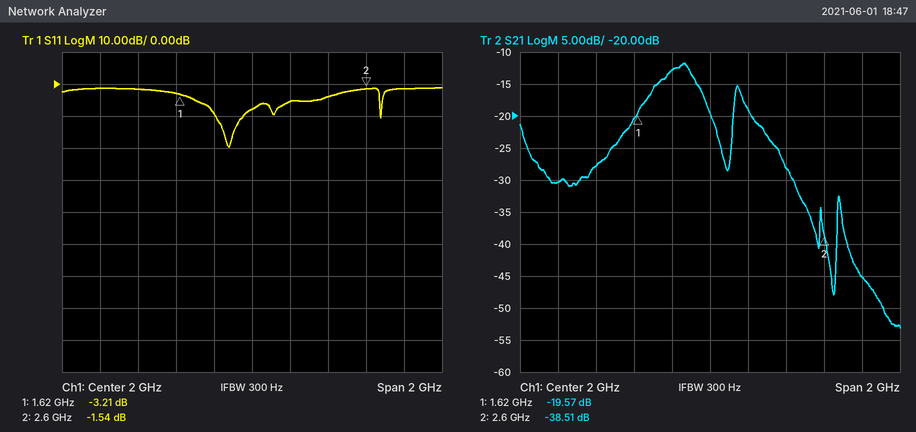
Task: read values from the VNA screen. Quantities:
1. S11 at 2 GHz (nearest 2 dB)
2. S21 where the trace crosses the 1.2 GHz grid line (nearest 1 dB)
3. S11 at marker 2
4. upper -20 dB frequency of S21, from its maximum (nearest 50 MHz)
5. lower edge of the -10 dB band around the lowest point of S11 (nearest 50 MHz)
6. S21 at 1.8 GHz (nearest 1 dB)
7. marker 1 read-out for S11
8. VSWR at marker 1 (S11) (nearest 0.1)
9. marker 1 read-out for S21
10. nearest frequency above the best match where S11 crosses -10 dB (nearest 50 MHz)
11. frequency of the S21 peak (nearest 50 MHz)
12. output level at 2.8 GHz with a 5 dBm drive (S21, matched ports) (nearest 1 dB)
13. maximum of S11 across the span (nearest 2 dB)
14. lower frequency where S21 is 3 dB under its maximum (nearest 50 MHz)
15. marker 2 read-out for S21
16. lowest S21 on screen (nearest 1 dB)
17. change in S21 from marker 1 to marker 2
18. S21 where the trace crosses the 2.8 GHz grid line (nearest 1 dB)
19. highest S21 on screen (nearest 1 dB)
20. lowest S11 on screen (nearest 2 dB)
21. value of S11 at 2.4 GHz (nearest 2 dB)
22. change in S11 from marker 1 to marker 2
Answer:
-8 dB
-30 dB
-1.54 dB
2.45 GHz
1.80 GHz
-13 dB
-3.21 dB
5.5
-19.57 dB
1.95 GHz
1.85 GHz
-40 dBm
-2 dB
1.75 GHz
-38.51 dB
-53 dB
-18.94 dB
-45 dB
-12 dB
-20 dB
-4 dB
1.67 dB
